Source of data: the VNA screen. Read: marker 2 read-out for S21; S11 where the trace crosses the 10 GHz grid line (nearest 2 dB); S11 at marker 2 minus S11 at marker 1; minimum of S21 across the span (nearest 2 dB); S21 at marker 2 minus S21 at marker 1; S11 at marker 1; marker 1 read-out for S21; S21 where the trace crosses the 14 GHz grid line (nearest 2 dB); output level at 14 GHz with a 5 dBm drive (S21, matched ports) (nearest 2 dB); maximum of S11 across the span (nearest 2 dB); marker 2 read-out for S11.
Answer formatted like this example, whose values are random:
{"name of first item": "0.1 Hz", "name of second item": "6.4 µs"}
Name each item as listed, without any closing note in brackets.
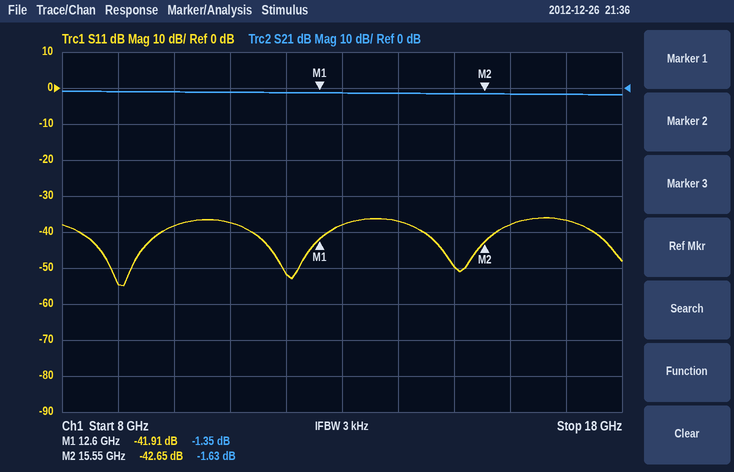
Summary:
{"marker 2 read-out for S21": "-1.63 dB", "S11 where the trace crosses the 10 GHz grid line": "-38 dB", "S11 at marker 2 minus S11 at marker 1": "-0.74 dB", "minimum of S21 across the span": "-2 dB", "S21 at marker 2 minus S21 at marker 1": "-0.28 dB", "S11 at marker 1": "-41.91 dB", "marker 1 read-out for S21": "-1.35 dB", "S21 where the trace crosses the 14 GHz grid line": "-2 dB", "output level at 14 GHz with a 5 dBm drive (S21, matched ports)": "4 dBm", "maximum of S11 across the span": "-36 dB", "marker 2 read-out for S11": "-42.65 dB"}
